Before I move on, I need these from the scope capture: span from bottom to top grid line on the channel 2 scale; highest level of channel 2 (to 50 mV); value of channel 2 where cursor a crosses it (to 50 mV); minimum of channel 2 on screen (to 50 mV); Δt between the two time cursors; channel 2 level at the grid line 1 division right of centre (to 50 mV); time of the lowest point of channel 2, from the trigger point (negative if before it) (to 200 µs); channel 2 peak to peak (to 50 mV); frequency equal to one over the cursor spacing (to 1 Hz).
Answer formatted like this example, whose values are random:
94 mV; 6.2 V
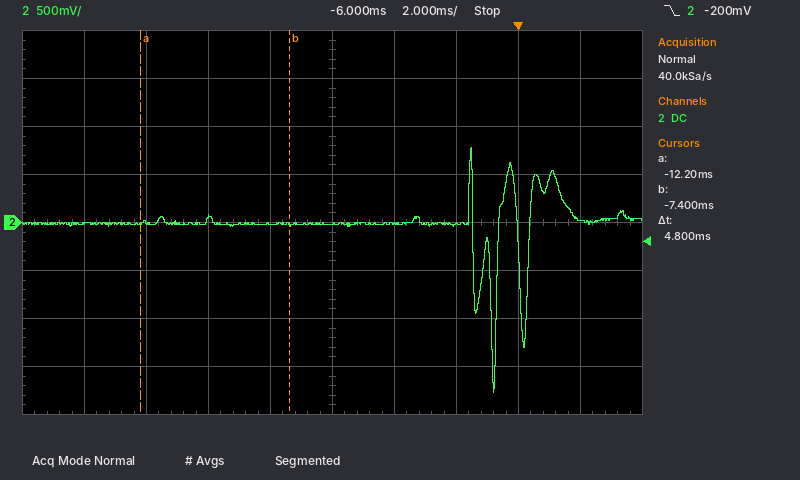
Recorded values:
4 V; 800 mV; 0 mV; -1.75 V; 4.8 ms; 0 mV; -800 µs; 2.55 V; 208 Hz
